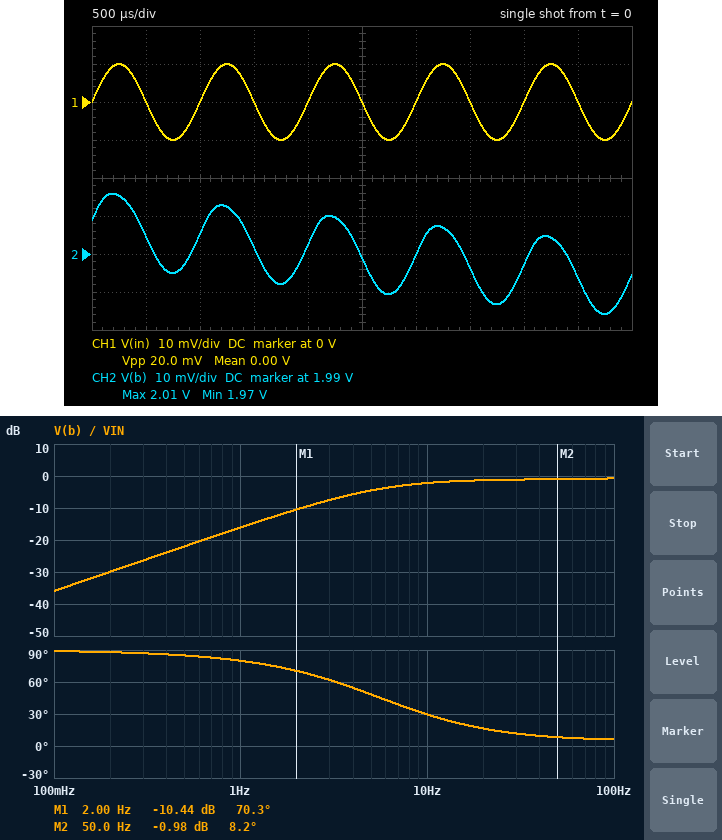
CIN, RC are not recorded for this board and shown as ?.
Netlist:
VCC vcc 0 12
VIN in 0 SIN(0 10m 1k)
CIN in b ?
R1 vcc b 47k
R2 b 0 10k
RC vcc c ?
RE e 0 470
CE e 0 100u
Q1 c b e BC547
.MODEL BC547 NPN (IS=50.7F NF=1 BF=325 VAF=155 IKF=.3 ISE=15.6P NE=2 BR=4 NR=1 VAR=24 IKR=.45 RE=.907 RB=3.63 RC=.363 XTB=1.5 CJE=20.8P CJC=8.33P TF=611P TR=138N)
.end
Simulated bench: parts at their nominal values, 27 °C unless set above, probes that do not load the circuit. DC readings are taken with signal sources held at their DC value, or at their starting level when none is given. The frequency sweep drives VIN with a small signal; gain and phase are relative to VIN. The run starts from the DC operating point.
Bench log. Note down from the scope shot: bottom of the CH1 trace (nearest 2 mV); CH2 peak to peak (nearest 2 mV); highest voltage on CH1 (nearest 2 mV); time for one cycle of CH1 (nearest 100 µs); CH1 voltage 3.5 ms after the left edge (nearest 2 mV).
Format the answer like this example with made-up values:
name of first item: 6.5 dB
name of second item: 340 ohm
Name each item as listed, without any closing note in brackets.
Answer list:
bottom of the CH1 trace: -10 mV
CH2 peak to peak: 32 mV
highest voltage on CH1: 10 mV
time for one cycle of CH1: 1.0 ms
CH1 voltage 3.5 ms after the left edge: 0 V
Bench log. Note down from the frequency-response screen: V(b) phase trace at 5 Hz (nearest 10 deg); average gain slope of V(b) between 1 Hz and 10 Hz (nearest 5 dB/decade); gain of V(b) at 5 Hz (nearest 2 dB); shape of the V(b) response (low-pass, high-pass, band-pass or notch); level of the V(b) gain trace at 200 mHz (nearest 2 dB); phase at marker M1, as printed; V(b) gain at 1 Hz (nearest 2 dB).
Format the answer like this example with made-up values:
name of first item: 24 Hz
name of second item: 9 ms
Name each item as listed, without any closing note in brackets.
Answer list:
V(b) phase trace at 5 Hz: 50 deg
average gain slope of V(b) between 1 Hz and 10 Hz: 15 dB/decade
gain of V(b) at 5 Hz: -4 dB
shape of the V(b) response: high-pass
level of the V(b) gain trace at 200 mHz: -30 dB
phase at marker M1, as printed: 70.3 deg
V(b) gain at 1 Hz: -16 dB
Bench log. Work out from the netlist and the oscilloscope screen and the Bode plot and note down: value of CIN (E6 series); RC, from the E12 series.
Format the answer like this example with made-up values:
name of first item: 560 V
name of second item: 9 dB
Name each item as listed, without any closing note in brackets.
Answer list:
value of CIN: 3.3 µF
RC, from the E12 series: 3.3 kΩ
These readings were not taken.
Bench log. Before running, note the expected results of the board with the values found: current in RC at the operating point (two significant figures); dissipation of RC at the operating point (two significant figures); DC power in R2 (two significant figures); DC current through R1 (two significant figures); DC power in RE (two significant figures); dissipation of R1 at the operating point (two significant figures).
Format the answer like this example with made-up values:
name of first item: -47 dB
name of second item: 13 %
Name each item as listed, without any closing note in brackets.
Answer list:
current in RC at the operating point: 2.9 mA
dissipation of RC at the operating point: 27 mW
DC power in R2: 400 µW
DC current through R1: 210 µA
DC power in RE: 3.9 mW
dissipation of R1 at the operating point: 2.1 mW
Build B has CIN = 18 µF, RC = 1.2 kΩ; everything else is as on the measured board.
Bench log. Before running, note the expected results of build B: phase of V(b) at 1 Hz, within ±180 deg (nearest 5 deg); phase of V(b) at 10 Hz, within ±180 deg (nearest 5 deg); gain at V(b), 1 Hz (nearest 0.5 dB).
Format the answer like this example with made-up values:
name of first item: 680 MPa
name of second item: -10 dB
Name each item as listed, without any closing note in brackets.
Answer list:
phase of V(b) at 1 Hz, within ±180 deg: 50 deg
phase of V(b) at 10 Hz, within ±180 deg: 5 deg
gain at V(b), 1 Hz: -3.5 dB
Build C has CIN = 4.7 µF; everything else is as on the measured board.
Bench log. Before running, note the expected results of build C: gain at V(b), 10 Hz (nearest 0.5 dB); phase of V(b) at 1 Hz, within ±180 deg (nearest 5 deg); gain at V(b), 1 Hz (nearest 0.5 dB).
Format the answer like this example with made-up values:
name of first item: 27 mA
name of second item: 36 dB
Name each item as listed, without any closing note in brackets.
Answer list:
gain at V(b), 10 Hz: -1.5 dB
phase of V(b) at 1 Hz, within ±180 deg: 75 deg
gain at V(b), 1 Hz: -13.0 dB
